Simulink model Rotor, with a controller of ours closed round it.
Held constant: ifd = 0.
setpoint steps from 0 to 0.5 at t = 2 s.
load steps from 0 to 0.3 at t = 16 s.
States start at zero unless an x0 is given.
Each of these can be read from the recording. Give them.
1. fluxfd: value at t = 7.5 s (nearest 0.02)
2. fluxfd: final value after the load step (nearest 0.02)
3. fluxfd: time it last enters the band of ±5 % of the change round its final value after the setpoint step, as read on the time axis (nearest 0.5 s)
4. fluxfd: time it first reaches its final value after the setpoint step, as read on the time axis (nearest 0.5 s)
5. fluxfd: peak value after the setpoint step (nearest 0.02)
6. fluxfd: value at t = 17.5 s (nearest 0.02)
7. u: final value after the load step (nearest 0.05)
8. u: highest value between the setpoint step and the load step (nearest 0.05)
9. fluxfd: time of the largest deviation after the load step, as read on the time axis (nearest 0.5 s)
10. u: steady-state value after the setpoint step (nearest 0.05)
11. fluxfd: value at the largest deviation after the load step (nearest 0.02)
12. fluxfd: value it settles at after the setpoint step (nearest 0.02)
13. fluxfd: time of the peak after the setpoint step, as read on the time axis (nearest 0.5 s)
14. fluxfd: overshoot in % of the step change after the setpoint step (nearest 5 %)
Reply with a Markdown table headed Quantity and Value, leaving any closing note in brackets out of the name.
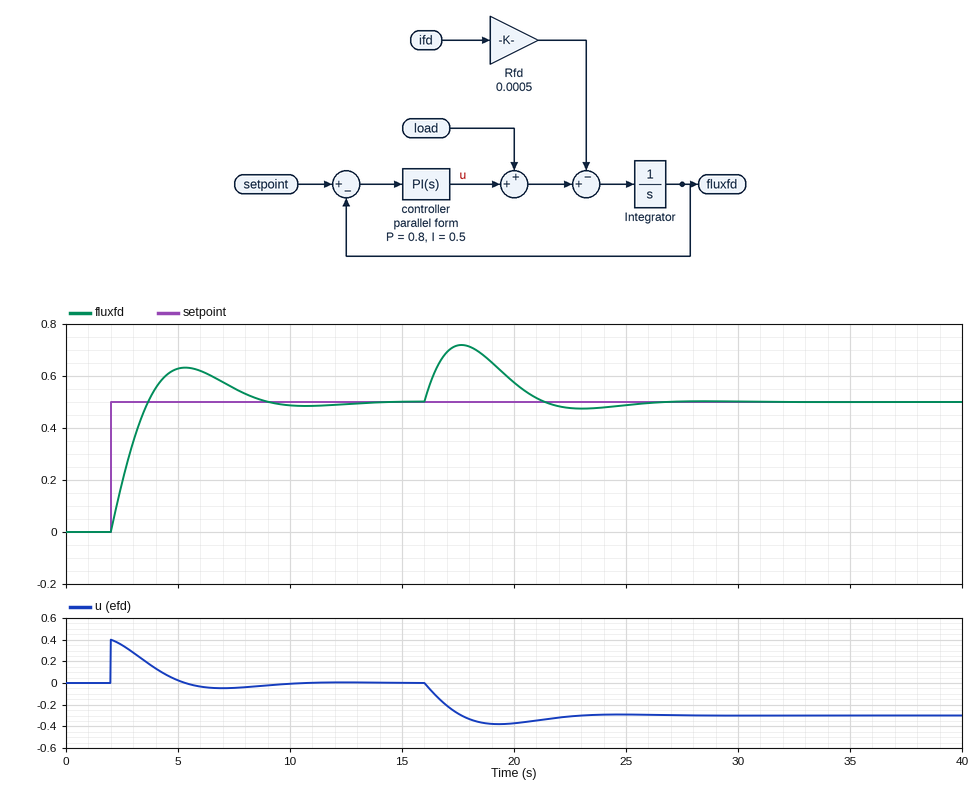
| Quantity | Value |
|---|---|
| fluxfd: value at t = 7.5 s | 0.56 |
| fluxfd: final value after the load step | 0.50 |
| fluxfd: time it last enters the band of ±5 % of the change round its final value after the setpoint step, as read on the time axis | 8.0 s |
| fluxfd: time it first reaches its final value after the setpoint step, as read on the time axis | 3.5 s |
| fluxfd: peak value after the setpoint step | 0.64 |
| fluxfd: value at t = 17.5 s | 0.72 |
| u: final value after the load step | -0.30 |
| u: highest value between the setpoint step and the load step | 0.40 |
| fluxfd: time of the largest deviation after the load step, as read on the time axis | 17.5 s |
| u: steady-state value after the setpoint step | 0.00 |
| fluxfd: value at the largest deviation after the load step | 0.72 |
| fluxfd: value it settles at after the setpoint step | 0.50 |
| fluxfd: time of the peak after the setpoint step, as read on the time axis | 5.5 s |
| fluxfd: overshoot in % of the step change after the setpoint step | 25 % |
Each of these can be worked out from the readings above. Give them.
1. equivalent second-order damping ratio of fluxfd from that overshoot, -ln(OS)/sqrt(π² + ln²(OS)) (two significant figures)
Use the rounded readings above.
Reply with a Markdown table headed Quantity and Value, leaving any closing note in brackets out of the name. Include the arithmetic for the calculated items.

| Quantity | Value |
|---|---|
| equivalent second-order damping ratio of fluxfd from that overshoot, -ln(OS)/sqrt(π² + ln²(OS)) | ln(0.25) = -1.386; 1.386 / sqrt(9.870 + 1.922) = 0.40 |
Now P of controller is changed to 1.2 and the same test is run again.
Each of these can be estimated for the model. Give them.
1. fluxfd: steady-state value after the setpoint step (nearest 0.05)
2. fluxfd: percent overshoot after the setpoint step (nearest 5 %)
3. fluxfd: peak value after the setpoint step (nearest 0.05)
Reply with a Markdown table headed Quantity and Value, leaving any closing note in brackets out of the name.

| Quantity | Value |
|---|---|
| fluxfd: steady-state value after the setpoint step | 0.50 |
| fluxfd: percent overshoot after the setpoint step | 15 % |
| fluxfd: peak value after the setpoint step | 0.60 |
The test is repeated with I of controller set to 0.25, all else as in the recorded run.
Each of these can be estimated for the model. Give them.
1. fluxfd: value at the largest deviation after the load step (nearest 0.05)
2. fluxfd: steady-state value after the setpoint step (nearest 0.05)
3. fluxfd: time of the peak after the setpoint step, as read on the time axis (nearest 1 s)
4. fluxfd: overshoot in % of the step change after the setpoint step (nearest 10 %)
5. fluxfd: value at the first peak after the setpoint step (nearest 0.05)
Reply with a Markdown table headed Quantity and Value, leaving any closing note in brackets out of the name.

| Quantity | Value |
|---|---|
| fluxfd: value at the largest deviation after the load step | 0.75 |
| fluxfd: steady-state value after the setpoint step | 0.50 |
| fluxfd: time of the peak after the setpoint step, as read on the time axis | 6 s |
| fluxfd: overshoot in % of the step change after the setpoint step | 20 % |
| fluxfd: value at the first peak after the setpoint step | 0.60 |
